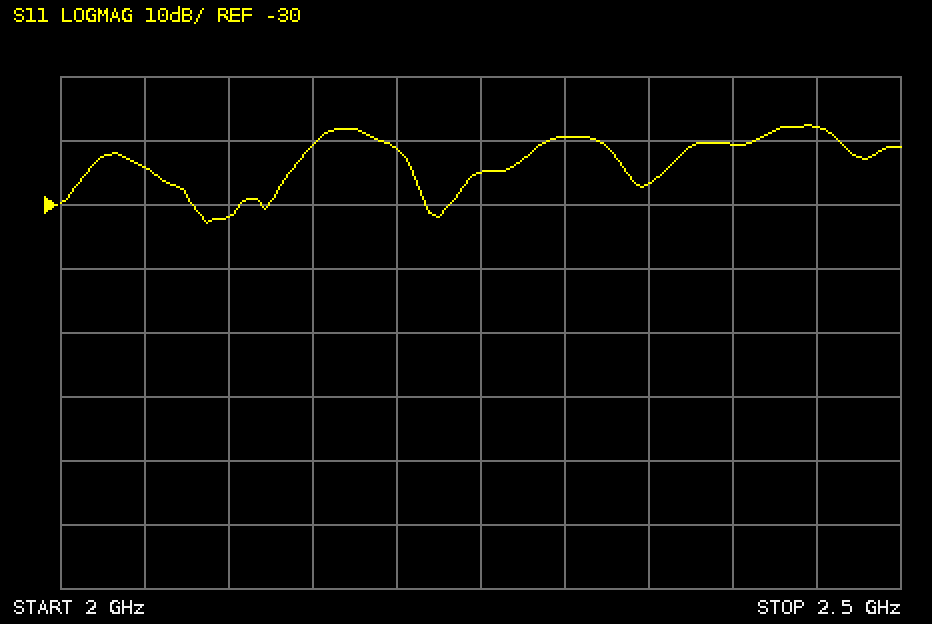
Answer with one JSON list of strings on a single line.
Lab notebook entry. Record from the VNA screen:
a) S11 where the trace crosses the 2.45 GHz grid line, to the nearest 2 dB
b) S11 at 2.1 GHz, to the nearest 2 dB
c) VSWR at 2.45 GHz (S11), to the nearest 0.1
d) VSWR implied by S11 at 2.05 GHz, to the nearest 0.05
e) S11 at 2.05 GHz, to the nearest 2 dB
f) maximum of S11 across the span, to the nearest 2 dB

["-18 dB", "-32 dB", "1.3", "1.15", "-24 dB", "-18 dB"]
